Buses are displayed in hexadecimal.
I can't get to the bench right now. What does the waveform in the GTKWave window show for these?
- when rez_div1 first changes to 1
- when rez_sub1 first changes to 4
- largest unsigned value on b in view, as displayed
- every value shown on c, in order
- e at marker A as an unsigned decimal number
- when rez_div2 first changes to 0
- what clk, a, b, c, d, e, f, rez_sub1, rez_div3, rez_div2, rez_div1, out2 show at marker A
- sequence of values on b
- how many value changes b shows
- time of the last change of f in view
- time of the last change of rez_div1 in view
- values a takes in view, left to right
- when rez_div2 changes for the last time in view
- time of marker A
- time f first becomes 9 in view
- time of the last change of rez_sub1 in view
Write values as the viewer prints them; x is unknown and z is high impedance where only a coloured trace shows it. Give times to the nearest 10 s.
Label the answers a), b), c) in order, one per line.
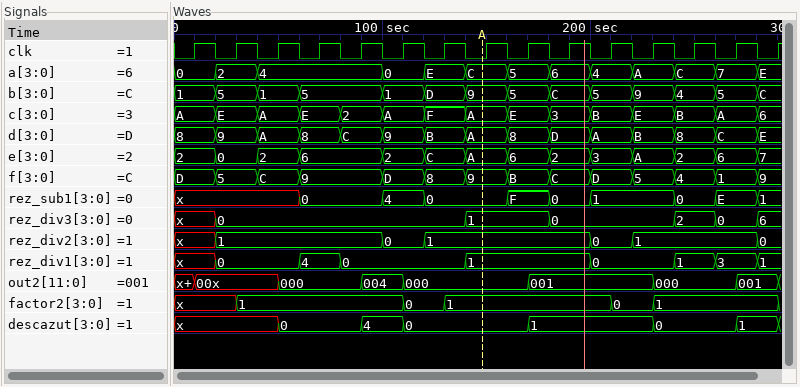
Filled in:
a) 140 s
b) 100 s
c) D
d) A, E, A, E, 2, A, F, A, E, 3, B, E, B, A, 6
e) 10
f) 100 s
g) clk=0, a=C, b=9, c=A, d=A, e=A, f=9, rez_sub1=0, rez_div3=1, rez_div2=1, rez_div1=1, out2=000
h) 1, 5, 1, 5, 1, D, 9, 5, C, 5, 9, 4, 5, C
i) 13
j) 280 s
k) 280 s
l) 0, 2, 4, 0, E, C, 5, 6, 4, A, C, 7, E
m) 280 s
n) 150 s
o) 60 s
p) 280 s
